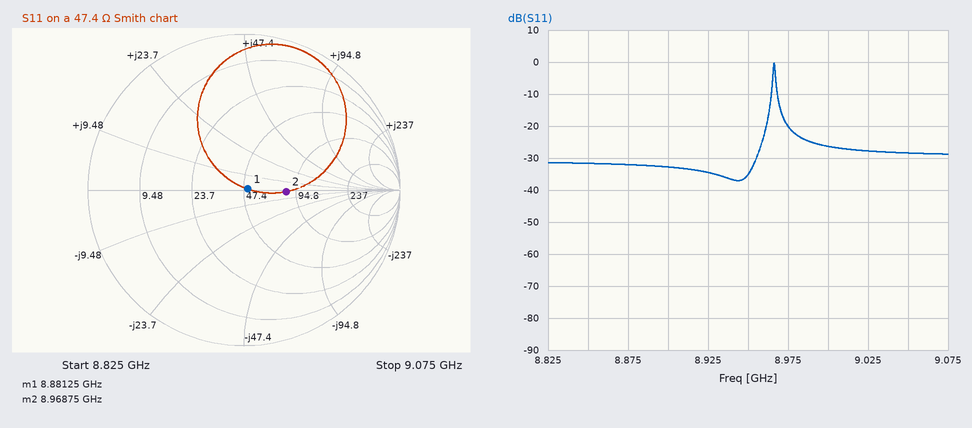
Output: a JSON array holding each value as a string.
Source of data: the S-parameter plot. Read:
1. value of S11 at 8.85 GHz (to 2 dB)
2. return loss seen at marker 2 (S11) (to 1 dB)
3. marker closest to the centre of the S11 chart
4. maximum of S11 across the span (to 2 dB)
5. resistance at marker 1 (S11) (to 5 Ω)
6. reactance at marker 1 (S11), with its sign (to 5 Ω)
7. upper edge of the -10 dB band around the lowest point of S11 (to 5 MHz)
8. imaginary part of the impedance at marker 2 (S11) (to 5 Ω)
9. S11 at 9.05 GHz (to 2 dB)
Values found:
["-32 dB", "11 dB", "marker 1", "0 dB", "50 Ω", "0 Ω", "8.965 GHz", "0 Ω", "-28 dB"]
